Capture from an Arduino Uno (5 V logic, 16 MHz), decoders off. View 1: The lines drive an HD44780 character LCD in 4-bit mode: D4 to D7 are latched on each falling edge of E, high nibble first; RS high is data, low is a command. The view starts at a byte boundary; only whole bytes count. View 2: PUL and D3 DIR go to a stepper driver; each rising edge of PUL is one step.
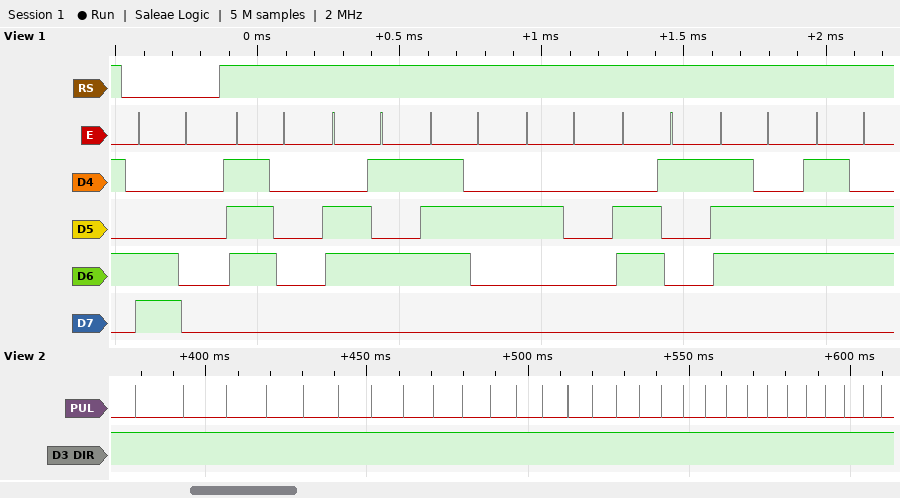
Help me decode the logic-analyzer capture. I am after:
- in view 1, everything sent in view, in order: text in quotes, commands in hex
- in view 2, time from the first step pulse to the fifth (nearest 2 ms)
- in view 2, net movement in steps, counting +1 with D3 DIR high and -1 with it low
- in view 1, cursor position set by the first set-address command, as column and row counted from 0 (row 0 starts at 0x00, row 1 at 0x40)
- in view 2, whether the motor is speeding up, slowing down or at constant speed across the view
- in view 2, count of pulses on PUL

0xC0 "per avv"
52 ms
+29
column 0, row 1
speeding up
29
